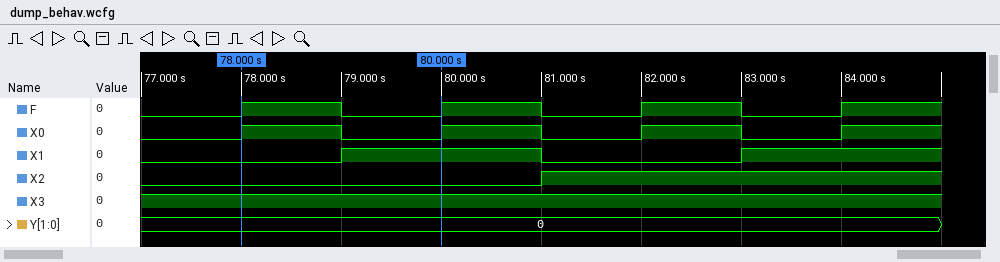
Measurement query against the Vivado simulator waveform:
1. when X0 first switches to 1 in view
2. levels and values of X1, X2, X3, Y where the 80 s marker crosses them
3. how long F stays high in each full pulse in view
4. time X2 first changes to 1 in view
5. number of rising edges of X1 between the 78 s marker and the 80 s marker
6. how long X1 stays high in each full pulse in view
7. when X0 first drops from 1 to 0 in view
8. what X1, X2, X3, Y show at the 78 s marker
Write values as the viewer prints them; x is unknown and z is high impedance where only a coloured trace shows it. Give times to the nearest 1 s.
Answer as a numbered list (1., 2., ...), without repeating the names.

1. 78 s
2. X1=1, X2=0, X3=1, Y=0
3. 1 s, 1 s, 1 s
4. 81 s
5. 1
6. 2 s
7. 79 s
8. X1=0, X2=0, X3=1, Y=0
